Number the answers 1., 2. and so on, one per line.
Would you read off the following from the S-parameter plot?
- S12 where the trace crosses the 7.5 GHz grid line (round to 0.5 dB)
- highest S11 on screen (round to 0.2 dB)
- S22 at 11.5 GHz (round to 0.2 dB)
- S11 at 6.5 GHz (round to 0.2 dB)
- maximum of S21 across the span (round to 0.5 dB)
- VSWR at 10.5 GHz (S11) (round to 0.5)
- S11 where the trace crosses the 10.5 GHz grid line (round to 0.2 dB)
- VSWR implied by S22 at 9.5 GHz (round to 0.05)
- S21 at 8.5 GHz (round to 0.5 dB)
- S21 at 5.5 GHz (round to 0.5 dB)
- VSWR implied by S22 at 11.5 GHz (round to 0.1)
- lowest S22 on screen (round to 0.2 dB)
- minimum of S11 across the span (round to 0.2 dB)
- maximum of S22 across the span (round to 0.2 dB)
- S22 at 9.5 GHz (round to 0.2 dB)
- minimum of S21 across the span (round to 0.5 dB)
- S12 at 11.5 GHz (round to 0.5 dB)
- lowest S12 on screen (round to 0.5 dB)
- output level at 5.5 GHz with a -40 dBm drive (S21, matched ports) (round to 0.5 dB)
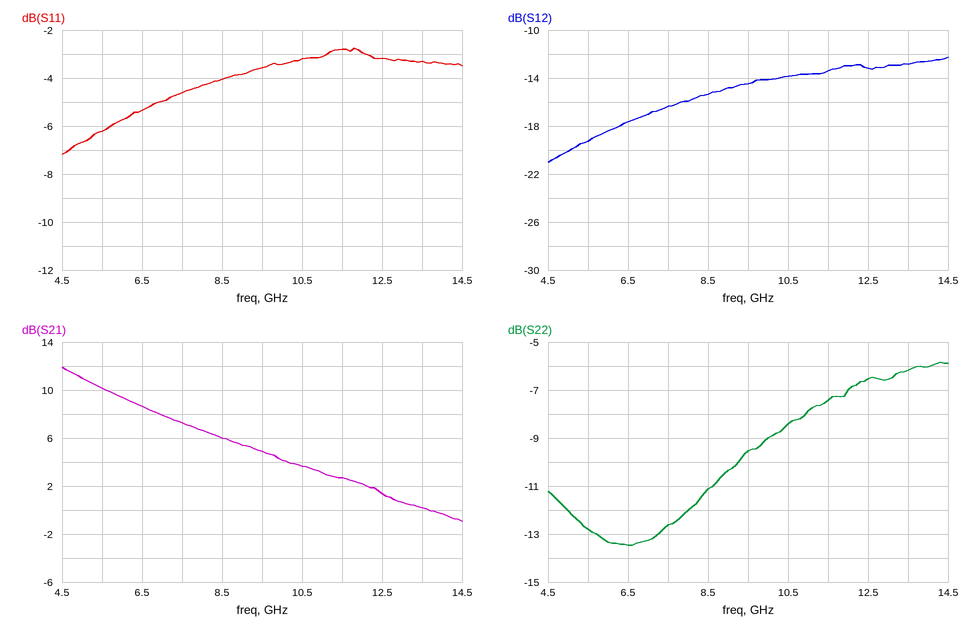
1. -16.5 dB
2. -2.8 dB
3. -7.4 dB
4. -5.4 dB
5. 12.0 dB
6. 5.5
7. -3.2 dB
8. 2.00
9. 6.0 dB
10. 10.0 dB
11. 2.5
12. -13.4 dB
13. -7.2 dB
14. -5.8 dB
15. -9.6 dB
16. -1.0 dB
17. -13.5 dB
18. -21.0 dB
19. -30.0 dBm
